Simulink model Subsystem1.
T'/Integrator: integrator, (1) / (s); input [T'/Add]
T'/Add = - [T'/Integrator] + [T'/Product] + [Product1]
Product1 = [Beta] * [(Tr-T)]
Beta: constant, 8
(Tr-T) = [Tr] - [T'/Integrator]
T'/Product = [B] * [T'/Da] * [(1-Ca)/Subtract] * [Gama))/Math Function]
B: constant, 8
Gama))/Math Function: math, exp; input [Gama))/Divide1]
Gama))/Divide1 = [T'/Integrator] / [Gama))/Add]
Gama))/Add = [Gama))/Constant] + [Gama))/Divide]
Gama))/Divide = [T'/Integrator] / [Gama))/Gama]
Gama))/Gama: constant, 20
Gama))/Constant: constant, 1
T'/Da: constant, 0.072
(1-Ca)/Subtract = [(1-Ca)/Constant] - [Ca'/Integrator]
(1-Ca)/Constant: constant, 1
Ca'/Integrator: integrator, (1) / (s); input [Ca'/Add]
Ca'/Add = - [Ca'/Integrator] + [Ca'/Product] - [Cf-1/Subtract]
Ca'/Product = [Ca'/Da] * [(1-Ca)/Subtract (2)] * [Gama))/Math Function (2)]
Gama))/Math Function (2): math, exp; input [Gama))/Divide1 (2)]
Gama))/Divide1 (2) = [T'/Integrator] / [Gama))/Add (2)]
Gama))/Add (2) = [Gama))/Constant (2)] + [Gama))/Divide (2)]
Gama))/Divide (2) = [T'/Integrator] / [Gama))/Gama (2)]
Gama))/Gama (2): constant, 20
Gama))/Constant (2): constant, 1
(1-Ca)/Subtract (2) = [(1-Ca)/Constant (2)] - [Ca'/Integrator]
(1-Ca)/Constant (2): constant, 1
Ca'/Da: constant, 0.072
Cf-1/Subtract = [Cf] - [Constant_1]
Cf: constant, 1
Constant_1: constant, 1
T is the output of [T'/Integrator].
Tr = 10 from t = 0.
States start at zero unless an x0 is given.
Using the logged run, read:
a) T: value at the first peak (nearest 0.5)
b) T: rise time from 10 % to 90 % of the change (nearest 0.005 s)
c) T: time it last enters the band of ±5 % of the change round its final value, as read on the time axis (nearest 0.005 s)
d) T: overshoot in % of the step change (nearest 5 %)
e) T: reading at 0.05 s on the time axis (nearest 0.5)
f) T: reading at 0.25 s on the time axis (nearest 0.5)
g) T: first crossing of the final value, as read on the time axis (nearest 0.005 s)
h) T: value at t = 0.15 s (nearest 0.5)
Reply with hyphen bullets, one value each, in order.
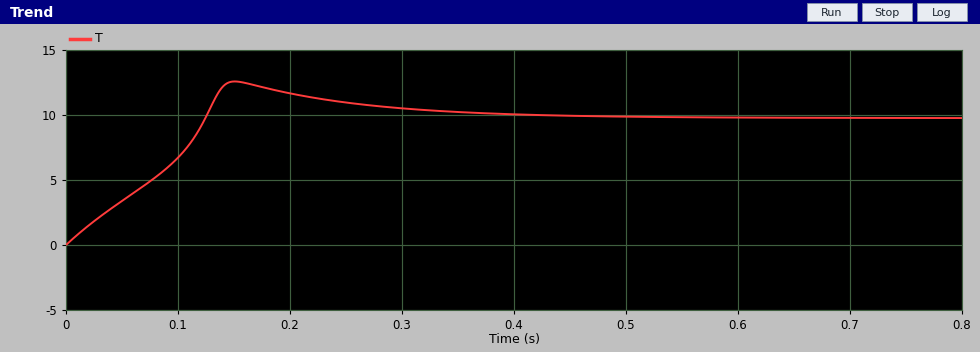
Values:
- 12.5
- 0.105 s
- 0.345 s
- 30 %
- 3.5
- 11.0
- 0.125 s
- 12.5
